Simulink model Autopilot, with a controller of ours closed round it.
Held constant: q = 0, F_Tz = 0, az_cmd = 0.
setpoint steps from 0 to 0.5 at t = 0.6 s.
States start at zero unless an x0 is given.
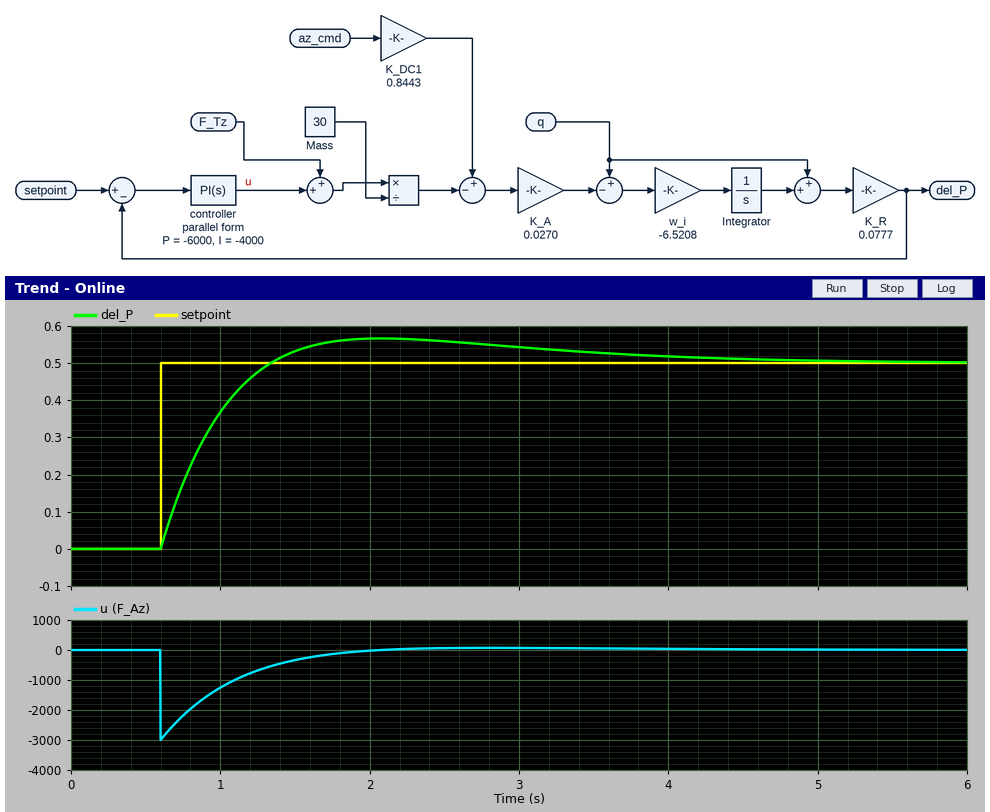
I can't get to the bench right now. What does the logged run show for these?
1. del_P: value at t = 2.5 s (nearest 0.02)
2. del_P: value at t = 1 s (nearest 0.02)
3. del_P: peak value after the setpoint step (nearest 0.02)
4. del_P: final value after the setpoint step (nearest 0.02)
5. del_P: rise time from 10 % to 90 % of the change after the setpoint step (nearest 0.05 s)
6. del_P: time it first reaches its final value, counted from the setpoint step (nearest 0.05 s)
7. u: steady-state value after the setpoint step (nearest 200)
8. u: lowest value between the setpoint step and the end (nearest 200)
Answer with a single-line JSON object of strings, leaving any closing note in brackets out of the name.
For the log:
{"del_P: value at t = 2.5 s": "0.56", "del_P: value at t = 1 s": "0.36", "del_P: peak value after the setpoint step": "0.56", "del_P: final value after the setpoint step": "0.50", "del_P: rise time from 10 % to 90 % of the change after the setpoint step": "0.55 s", "del_P: time it first reaches its final value, counted from the setpoint step": "0.75 s", "u: steady-state value after the setpoint step": "0", "u: lowest value between the setpoint step and the end": "-3000"}
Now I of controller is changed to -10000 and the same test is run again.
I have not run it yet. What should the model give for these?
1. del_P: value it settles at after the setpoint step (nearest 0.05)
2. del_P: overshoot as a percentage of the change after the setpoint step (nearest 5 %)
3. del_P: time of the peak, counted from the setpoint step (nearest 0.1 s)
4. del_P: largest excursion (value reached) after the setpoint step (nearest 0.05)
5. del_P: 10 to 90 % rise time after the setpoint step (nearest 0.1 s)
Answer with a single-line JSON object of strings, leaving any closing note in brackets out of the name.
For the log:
{"del_P: value it settles at after the setpoint step": "0.50", "del_P: overshoot as a percentage of the change after the setpoint step": "25 %", "del_P: time of the peak, counted from the setpoint step": "1.1 s", "del_P: largest excursion (value reached) after the setpoint step": "0.60", "del_P: 10 to 90 % rise time after the setpoint step": "0.4 s"}
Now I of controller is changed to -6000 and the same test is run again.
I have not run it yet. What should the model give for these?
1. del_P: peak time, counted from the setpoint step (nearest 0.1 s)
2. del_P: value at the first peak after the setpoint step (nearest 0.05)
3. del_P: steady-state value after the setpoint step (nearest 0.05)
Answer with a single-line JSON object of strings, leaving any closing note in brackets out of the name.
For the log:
{"del_P: peak time, counted from the setpoint step": "1.3 s", "del_P: value at the first peak after the setpoint step": "0.60", "del_P: steady-state value after the setpoint step": "0.50"}
